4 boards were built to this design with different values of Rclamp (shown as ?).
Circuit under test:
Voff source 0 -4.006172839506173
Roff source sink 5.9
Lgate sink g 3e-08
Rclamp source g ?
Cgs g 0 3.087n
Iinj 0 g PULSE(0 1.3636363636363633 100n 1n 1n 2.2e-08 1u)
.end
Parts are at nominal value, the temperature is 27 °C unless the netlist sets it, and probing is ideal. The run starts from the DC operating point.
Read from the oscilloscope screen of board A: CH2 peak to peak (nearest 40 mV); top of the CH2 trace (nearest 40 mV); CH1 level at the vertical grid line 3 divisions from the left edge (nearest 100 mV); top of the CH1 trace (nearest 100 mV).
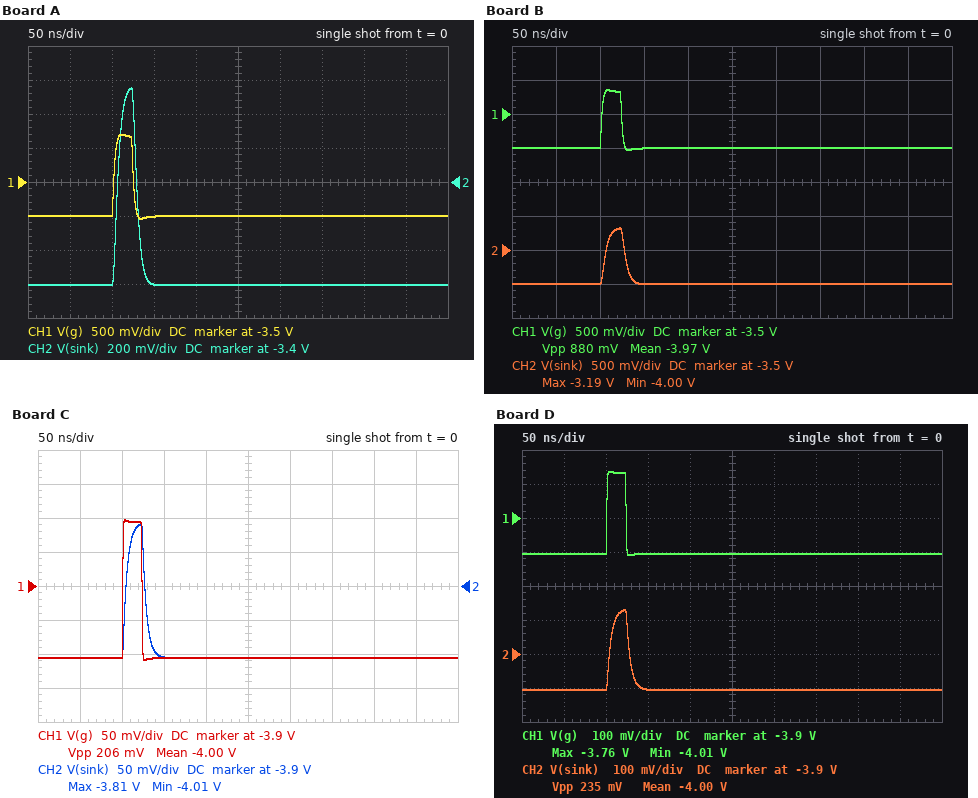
1.16 V
-2.84 V
-4.0 V
-2.8 V
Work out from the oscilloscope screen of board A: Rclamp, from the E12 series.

1 Ω
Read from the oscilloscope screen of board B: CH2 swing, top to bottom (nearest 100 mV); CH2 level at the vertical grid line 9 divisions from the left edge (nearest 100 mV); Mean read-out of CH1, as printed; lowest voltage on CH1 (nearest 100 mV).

800 mV
-4.0 V
-3.97 V
-4.0 V
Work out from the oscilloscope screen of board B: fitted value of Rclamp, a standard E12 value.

0.68 Ω
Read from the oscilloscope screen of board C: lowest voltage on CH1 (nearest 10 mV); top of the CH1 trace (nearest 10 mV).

-4.01 V
-3.80 V
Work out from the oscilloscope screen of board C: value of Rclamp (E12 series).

0.15 Ω
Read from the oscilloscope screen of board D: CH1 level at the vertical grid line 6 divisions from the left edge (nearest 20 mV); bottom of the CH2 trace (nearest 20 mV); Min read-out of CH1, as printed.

-4.00 V
-4.00 V
-4.01 V
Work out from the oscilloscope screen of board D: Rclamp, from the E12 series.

0.18 Ω
